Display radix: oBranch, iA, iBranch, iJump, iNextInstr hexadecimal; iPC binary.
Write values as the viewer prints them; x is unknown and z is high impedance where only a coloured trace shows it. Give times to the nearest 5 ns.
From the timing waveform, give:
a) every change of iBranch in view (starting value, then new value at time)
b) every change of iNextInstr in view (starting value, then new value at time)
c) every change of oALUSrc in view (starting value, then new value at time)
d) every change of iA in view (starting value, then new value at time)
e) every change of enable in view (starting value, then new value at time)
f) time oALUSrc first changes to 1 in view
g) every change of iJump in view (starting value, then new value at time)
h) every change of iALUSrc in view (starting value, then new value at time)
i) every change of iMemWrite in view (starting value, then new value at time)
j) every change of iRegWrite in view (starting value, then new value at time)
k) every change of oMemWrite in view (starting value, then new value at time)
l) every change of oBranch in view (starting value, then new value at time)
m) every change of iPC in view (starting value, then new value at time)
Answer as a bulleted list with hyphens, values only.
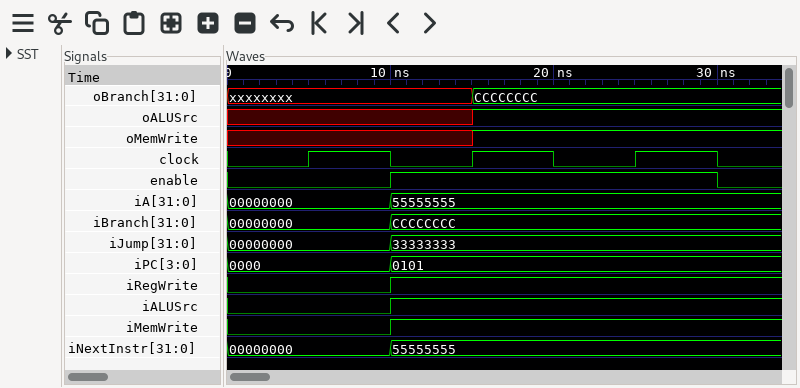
- 00000000, CCCCCCCC at 10 ns
- 00000000, 55555555 at 10 ns
- x, 1 at 15 ns
- 00000000, 55555555 at 10 ns
- 0, 1 at 10 ns, 0 at 30 ns
- 15 ns
- 00000000, 33333333 at 10 ns
- 0, 1 at 10 ns
- 0, 1 at 10 ns
- 0, 1 at 10 ns
- x, 1 at 15 ns
- xxxxxxxx, CCCCCCCC at 15 ns
- 0000, 0101 at 10 ns
